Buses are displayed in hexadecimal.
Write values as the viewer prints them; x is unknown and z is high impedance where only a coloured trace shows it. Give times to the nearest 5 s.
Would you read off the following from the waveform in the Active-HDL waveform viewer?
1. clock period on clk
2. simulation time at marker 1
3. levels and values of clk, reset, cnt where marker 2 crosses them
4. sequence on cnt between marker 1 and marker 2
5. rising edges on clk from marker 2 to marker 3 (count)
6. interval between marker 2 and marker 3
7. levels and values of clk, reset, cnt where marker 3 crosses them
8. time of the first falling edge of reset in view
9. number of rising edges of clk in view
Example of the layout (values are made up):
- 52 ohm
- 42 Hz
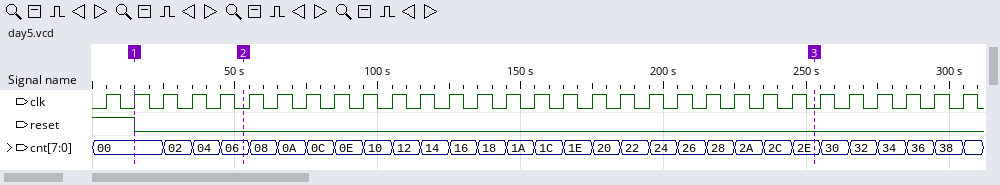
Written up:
- 10 s
- 15 s
- clk=0, reset=0, cnt=06
- 00, 02, 04, 06
- 20
- 200 s
- clk=0, reset=0, cnt=2E
- 15 s
- 31
